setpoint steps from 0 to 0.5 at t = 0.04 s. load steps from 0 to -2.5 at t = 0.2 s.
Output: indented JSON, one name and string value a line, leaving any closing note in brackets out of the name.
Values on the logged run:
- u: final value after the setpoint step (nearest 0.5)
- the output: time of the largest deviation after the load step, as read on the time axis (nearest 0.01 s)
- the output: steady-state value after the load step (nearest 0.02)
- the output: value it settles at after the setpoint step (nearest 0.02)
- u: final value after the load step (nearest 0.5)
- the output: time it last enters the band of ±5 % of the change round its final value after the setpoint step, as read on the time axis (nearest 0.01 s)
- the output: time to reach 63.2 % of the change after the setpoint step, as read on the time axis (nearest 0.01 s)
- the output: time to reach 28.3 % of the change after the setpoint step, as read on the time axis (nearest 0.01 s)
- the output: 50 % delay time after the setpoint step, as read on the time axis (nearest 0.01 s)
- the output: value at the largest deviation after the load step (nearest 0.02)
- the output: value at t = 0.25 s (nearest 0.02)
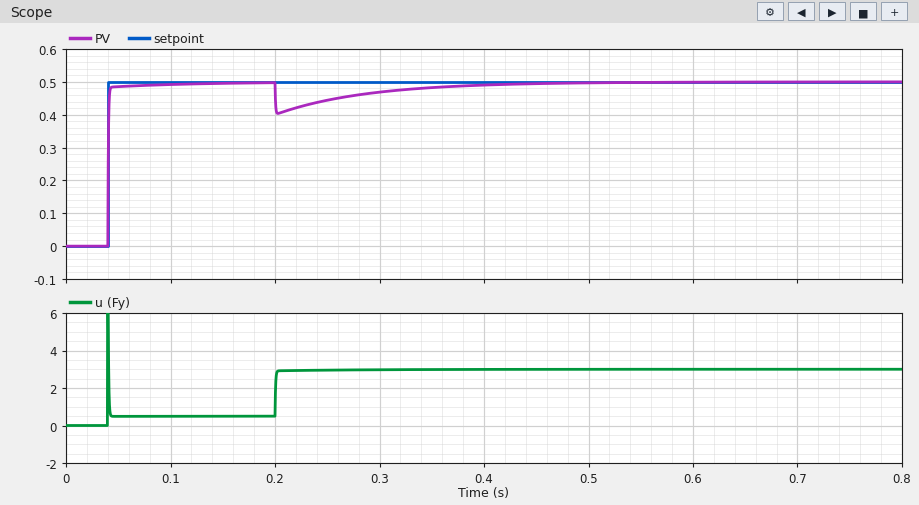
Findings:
{
  "u: final value after the setpoint step": "0.5",
  "the output: time of the largest deviation after the load step, as read on the time axis": "0.20 s",
  "the output: steady-state value after the load step": "0.50",
  "the output: value it settles at after the setpoint step": "0.50",
  "u: final value after the load step": "3.0",
  "the output: time it last enters the band of ±5 % of the change round its final value after the setpoint step, as read on the time axis": "0.04 s",
  "the output: time to reach 63.2 % of the change after the setpoint step, as read on the time axis": "0.04 s",
  "the output: time to reach 28.3 % of the change after the setpoint step, as read on the time axis": "0.04 s",
  "the output: 50 % delay time after the setpoint step, as read on the time axis": "0.04 s",
  "the output: value at the largest deviation after the load step": "0.40",
  "the output: value at t = 0.25 s": "0.44"
}
